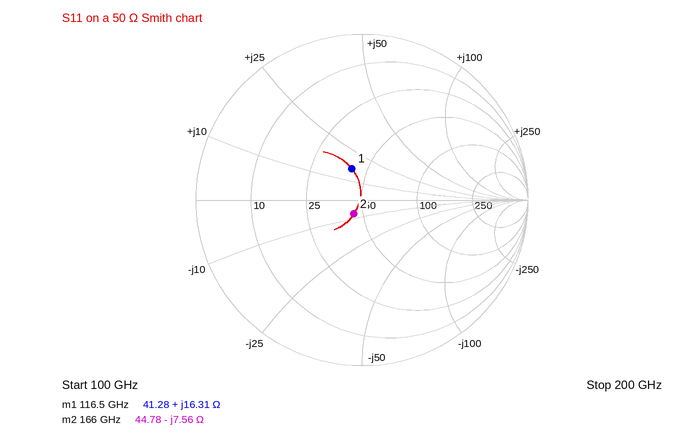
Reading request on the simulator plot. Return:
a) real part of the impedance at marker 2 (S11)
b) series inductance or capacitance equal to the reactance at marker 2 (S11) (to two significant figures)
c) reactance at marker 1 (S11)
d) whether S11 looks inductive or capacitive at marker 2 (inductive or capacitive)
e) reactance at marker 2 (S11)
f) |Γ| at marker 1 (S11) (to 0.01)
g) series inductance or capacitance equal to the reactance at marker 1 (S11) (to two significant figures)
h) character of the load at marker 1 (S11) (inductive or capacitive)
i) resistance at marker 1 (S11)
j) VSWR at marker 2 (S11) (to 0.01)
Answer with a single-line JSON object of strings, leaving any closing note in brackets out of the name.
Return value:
{"real part of the impedance at marker 2": "44.78 Ω", "series inductance or capacitance equal to the reactance at marker 2 (S11)": "130 fF", "reactance at marker 1": "+16.31 Ω", "whether S11 looks inductive or capacitive at marker 2": "capacitive", "reactance at marker 2": "-7.56 Ω", "|Γ| at marker 1 (S11)": "0.20", "series inductance or capacitance equal to the reactance at marker 1 (S11)": "22 pH", "character of the load at marker 1 (S11)": "inductive", "resistance at marker 1": "41.28 Ω", "VSWR at marker 2 (S11)": "1.21"}
